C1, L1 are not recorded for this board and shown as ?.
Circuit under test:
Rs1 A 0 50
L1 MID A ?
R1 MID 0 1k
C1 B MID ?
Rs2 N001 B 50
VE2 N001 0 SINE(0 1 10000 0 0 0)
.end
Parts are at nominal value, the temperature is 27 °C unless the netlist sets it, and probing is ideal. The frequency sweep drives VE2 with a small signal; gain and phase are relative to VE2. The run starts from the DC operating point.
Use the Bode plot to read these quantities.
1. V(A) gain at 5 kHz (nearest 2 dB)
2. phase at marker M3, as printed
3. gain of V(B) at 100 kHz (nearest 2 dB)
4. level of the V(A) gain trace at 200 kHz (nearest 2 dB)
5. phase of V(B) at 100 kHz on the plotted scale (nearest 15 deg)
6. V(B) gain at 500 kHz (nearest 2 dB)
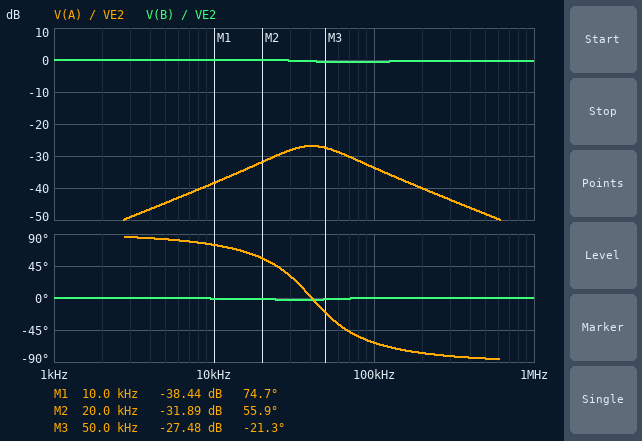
-44 dB
-21.3 deg
0 dB
-40 dB
0 deg
0 dB
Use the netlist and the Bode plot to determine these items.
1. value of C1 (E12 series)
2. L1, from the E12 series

3.9 nF
3.9 mH
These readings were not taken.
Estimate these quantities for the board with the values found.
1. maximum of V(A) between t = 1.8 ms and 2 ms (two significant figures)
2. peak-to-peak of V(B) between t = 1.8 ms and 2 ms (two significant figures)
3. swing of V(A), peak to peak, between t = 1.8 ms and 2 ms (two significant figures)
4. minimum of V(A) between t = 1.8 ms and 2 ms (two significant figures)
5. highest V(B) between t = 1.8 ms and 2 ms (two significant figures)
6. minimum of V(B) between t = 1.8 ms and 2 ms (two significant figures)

12 mV
2.0 V
24 mV
-12 mV
1.0 V
-1.0 V
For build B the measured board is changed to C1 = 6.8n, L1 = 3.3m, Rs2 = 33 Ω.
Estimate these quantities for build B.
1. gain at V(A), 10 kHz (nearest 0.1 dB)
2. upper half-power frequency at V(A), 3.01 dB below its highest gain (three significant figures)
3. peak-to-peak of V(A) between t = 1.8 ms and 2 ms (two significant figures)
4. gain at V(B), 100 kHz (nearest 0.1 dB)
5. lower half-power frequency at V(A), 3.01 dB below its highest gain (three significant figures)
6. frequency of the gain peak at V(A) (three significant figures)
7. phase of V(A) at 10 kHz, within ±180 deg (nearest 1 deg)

-33.3 dB
49.7 kHz
43 mV
-0.3 dB
23.1 kHz
33.9 kHz
76 deg
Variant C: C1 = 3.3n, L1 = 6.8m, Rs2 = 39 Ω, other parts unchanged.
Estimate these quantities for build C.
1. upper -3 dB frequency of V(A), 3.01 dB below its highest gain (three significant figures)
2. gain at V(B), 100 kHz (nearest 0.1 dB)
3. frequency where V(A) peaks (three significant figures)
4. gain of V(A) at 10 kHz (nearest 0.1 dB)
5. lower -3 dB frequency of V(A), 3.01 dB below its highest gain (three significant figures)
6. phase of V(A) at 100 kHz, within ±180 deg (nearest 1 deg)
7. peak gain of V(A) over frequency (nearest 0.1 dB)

65.8 kHz
-0.3 dB
33.8 kHz
-40.2 dB
17.3 kHz
-61 deg
-32.7 dB
